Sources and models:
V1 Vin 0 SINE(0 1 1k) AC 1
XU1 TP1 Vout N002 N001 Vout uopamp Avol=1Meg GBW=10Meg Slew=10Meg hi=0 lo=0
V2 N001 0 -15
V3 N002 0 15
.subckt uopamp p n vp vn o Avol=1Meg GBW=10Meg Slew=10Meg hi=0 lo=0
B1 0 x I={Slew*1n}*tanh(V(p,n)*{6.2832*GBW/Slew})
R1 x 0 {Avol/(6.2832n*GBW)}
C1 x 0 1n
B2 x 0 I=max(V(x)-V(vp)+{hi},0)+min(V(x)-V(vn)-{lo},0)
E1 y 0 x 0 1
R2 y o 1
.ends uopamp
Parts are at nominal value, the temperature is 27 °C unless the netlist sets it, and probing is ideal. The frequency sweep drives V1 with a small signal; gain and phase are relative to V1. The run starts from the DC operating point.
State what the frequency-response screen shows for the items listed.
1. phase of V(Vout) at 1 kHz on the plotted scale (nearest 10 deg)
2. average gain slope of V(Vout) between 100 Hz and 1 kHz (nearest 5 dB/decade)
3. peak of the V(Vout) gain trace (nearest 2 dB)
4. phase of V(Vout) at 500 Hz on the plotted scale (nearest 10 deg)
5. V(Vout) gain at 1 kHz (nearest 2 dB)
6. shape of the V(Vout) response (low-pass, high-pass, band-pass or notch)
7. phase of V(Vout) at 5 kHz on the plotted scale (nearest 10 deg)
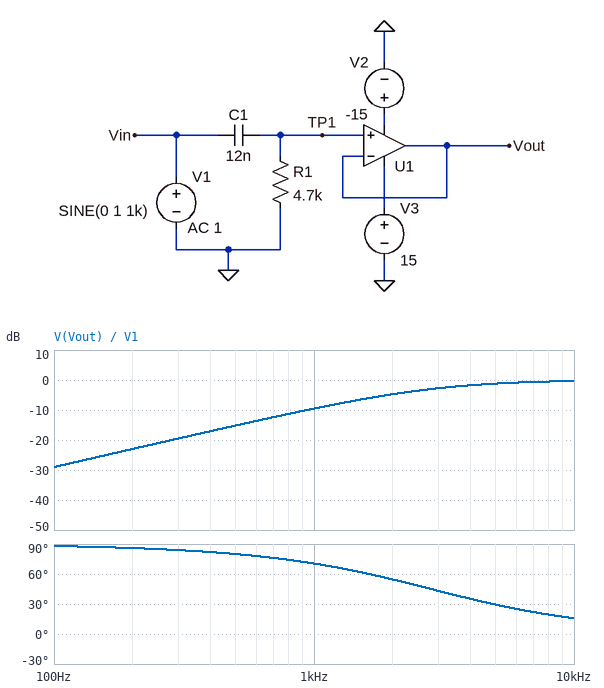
70 deg
20 dB/decade
0 dB
80 deg
-10 dB
high-pass
30 deg
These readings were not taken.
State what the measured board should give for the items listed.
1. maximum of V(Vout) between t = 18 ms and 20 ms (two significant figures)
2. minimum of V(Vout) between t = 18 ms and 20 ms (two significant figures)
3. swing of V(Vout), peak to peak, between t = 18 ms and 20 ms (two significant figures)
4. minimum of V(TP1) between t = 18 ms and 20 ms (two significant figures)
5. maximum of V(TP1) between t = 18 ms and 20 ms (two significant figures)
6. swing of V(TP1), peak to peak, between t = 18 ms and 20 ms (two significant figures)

330 mV
-330 mV
670 mV
-330 mV
330 mV
670 mV
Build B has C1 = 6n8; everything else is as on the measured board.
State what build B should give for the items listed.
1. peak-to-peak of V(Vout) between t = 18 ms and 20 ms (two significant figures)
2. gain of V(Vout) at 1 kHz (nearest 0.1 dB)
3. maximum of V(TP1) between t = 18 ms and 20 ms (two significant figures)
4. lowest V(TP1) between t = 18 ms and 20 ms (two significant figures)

390 mV
-14.1 dB
200 mV
-200 mV
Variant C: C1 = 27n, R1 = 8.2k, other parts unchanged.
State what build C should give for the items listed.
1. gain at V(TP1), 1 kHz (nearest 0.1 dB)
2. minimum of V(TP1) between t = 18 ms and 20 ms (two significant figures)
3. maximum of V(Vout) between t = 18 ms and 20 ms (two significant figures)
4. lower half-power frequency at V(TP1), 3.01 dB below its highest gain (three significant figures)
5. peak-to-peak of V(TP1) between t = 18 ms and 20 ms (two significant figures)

-1.8 dB
-810 mV
810 mV
719 Hz
1.6 V
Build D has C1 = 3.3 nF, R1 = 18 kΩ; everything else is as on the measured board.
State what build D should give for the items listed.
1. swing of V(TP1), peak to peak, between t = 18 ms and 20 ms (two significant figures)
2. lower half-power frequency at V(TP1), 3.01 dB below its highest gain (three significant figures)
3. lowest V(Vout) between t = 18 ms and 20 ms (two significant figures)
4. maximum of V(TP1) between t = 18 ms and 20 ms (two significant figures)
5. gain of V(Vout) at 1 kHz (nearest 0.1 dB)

700 mV
2.68 kHz
-350 mV
350 mV
-9.1 dB
